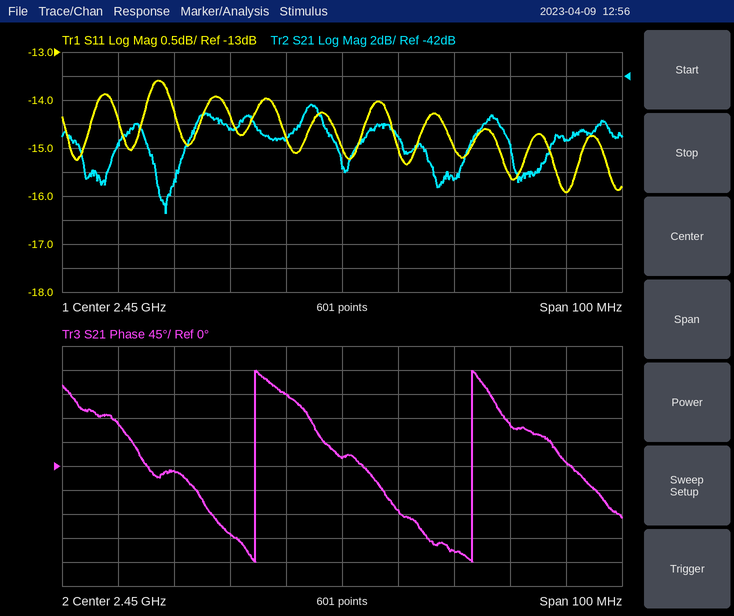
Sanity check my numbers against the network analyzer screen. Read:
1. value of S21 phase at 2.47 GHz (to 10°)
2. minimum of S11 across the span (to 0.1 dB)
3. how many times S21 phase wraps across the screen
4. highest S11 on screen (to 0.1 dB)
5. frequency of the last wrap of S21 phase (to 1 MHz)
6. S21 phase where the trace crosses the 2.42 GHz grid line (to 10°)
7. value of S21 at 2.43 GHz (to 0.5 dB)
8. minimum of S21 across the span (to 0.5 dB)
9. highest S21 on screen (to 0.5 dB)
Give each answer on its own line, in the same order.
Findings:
-160°
-15.9 dB
2
-13.6 dB
2.473 GHz
-10°
-46.5 dB
-53.5 dB
-44.5 dB
